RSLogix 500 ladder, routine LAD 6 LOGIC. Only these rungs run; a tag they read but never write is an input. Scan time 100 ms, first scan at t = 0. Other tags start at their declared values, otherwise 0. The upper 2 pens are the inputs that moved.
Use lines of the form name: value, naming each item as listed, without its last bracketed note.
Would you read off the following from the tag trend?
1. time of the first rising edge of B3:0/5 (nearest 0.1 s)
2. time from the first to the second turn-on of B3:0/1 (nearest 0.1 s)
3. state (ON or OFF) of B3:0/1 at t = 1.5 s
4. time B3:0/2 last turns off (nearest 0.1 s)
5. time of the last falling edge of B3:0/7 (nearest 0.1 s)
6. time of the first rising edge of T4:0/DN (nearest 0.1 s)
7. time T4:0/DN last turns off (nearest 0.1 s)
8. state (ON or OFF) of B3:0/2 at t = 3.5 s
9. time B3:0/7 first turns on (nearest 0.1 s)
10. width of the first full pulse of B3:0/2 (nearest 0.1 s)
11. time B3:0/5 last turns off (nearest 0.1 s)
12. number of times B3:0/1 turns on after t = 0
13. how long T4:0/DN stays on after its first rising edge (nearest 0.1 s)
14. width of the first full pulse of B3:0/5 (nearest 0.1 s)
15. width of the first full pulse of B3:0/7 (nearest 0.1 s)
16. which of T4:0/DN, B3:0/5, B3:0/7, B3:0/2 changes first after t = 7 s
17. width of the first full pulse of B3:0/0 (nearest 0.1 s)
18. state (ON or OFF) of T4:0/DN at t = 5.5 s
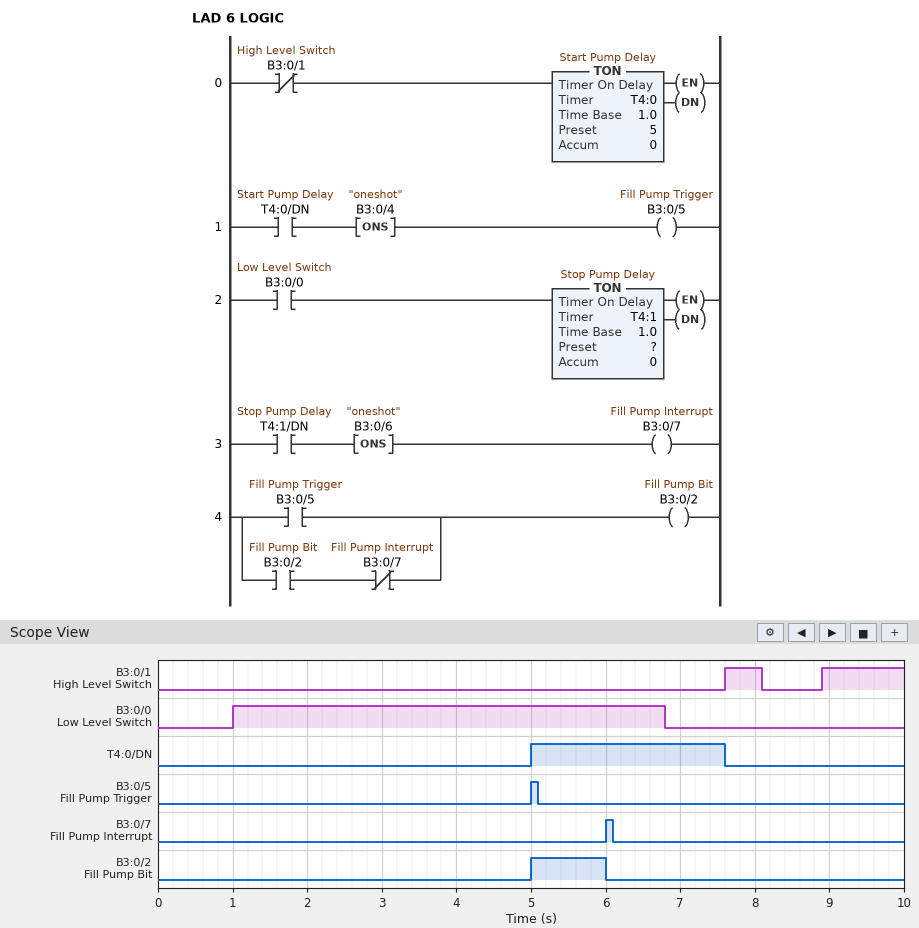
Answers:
time of the first rising edge of B3:0/5: 5.0 s
time from the first to the second turn-on of B3:0/1: 1.3 s
state (ON or OFF) of B3:0/1 at t = 1.5 s: OFF
time B3:0/2 last turns off: 6.0 s
time of the last falling edge of B3:0/7: 6.1 s
time of the first rising edge of T4:0/DN: 5.0 s
time T4:0/DN last turns off: 7.6 s
state (ON or OFF) of B3:0/2 at t = 3.5 s: OFF
time B3:0/7 first turns on: 6.0 s
width of the first full pulse of B3:0/2: 1.0 s
time B3:0/5 last turns off: 5.1 s
number of times B3:0/1 turns on after t = 0: 2
how long T4:0/DN stays on after its first rising edge: 2.6 s
width of the first full pulse of B3:0/5: 0.1 s
width of the first full pulse of B3:0/7: 0.1 s
which of T4:0/DN, B3:0/5, B3:0/7, B3:0/2 changes first after t = 7 s: T4:0/DN
width of the first full pulse of B3:0/0: 5.8 s
state (ON or OFF) of T4:0/DN at t = 5.5 s: ON
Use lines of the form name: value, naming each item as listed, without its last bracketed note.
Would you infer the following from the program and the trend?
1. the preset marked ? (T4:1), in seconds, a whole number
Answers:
the preset marked ? (T4:1), in seconds, a whole number: 5 s
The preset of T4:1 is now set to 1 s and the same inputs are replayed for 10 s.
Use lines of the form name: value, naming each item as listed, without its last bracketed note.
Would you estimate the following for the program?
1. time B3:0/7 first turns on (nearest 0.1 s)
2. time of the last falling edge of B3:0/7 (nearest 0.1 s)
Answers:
time B3:0/7 first turns on: 2.0 s
time of the last falling edge of B3:0/7: 2.1 s
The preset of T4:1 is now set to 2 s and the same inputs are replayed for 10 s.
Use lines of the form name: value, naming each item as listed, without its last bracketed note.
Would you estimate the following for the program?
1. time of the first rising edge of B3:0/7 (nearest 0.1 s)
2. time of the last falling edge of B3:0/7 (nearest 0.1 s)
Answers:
time of the first rising edge of B3:0/7: 3.0 s
time of the last falling edge of B3:0/7: 3.1 s
